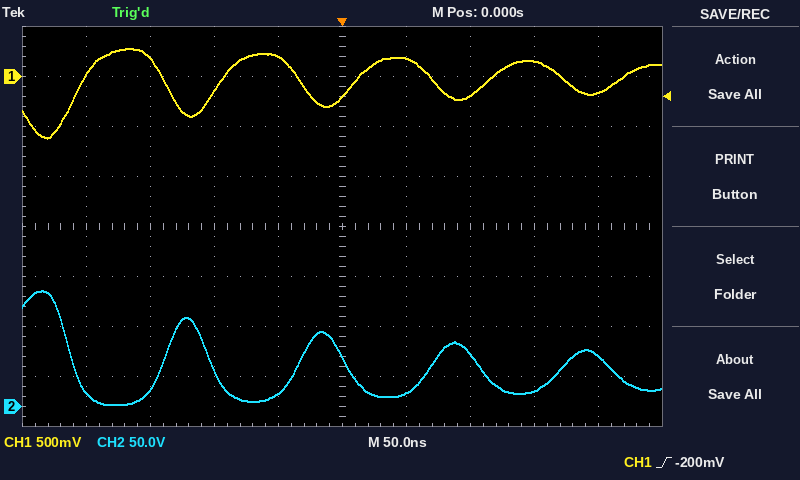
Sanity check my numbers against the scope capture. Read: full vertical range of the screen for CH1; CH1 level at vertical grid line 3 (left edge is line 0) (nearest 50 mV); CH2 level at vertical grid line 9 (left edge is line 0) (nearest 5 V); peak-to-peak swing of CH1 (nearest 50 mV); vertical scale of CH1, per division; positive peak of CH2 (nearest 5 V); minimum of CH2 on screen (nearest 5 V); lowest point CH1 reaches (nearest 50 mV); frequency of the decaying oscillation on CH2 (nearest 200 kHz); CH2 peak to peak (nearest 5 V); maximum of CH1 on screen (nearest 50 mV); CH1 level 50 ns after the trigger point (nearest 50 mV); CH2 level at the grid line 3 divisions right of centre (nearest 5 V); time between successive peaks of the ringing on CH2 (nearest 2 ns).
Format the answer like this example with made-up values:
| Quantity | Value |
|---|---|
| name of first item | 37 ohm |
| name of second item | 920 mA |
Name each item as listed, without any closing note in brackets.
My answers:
| Quantity | Value |
|---|---|
| full vertical range of the screen for CH1 | 4 V |
| CH1 level at vertical grid line 3 (left edge is line 0) | -150 mV |
| CH2 level at vertical grid line 9 (left edge is line 0) | 50 V |
| peak-to-peak swing of CH1 | 900 mV |
| vertical scale of CH1, per division | 500 mV |
| positive peak of CH2 | 115 V |
| minimum of CH2 on screen | 0 V |
| lowest point CH1 reaches | -600 mV |
| frequency of the decaying oscillation on CH2 | 9.4 MHz |
| CH2 peak to peak | 115 V |
| maximum of CH1 on screen | 300 mV |
| CH1 level 50 ns after the trigger point | 200 mV |
| CH2 level at the grid line 3 divisions right of centre | 15 V |
| time between successive peaks of the ringing on CH2 | 106 ns |
